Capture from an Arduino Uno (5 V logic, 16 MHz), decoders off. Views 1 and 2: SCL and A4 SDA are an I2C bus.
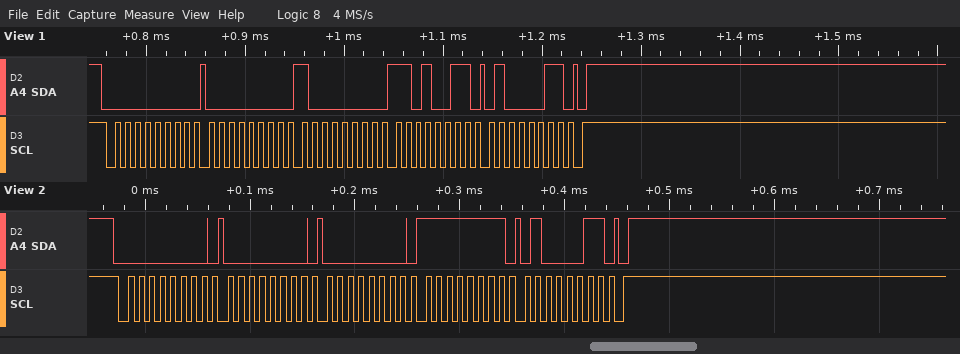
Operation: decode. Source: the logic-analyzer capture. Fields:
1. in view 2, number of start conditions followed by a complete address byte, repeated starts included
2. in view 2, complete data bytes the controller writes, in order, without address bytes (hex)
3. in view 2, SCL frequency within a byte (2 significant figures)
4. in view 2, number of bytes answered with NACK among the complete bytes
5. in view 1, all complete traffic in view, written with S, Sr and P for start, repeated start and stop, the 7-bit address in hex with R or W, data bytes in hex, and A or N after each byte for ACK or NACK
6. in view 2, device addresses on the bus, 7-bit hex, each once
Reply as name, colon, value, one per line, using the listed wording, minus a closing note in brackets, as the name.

in view 2, number of start conditions followed by a complete address byte, repeated starts included: 1
in view 2, complete data bytes the controller writes, in order, without address bytes: 00 00 FF 43
in view 2, SCL frequency within a byte: 100 kHz
in view 2, number of bytes answered with NACK among the complete bytes: 0
in view 1, all complete traffic in view, written with S, Sr and P for start, repeated start and stop, the 7-bit address in hex with R or W, data bytes in hex, and A or N after each byte for ACK or NACK: S 00W A 00 A 80 A D3 A 43 A P
in view 2, device addresses on the bus, 7-bit hex, each once: 0x00
